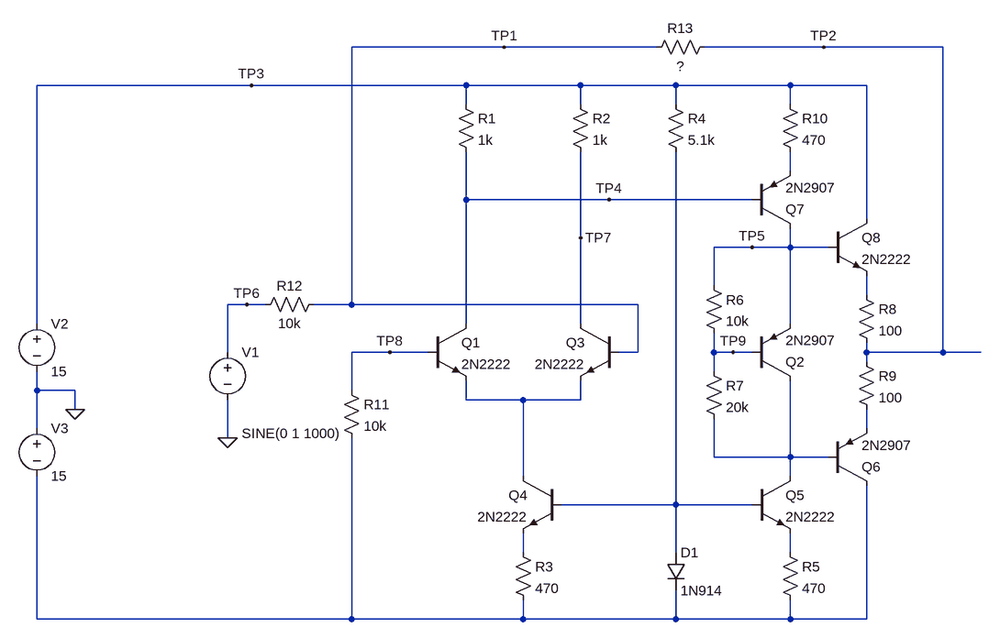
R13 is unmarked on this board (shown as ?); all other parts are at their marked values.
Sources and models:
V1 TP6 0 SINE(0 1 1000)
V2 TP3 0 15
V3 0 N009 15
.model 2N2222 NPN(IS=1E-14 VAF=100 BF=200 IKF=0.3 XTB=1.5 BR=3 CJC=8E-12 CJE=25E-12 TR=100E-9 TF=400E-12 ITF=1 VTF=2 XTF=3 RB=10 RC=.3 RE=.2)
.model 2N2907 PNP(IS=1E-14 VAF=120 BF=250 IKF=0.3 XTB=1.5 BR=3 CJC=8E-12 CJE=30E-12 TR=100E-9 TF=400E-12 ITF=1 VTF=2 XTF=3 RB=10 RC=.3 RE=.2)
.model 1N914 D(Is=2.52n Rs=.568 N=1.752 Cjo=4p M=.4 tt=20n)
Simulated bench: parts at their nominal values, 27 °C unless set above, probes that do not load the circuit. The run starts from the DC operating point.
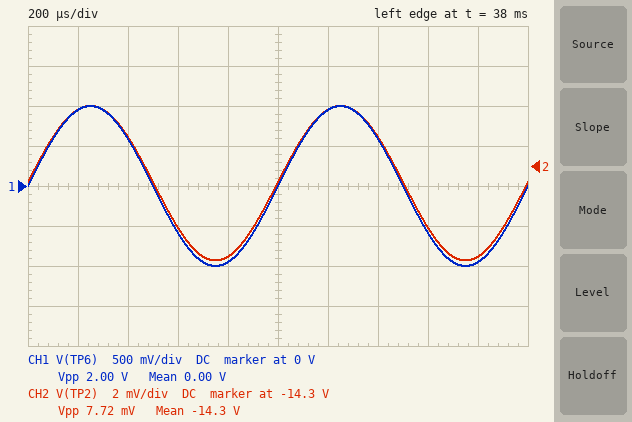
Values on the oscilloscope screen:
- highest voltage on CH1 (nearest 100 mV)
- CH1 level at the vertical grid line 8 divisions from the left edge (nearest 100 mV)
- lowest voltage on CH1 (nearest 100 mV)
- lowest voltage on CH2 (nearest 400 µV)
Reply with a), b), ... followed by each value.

a) 1.0 V
b) -600 mV
c) -1.0 V
d) -14.3048 V
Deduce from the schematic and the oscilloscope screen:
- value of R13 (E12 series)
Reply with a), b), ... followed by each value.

a) 39 kΩ
